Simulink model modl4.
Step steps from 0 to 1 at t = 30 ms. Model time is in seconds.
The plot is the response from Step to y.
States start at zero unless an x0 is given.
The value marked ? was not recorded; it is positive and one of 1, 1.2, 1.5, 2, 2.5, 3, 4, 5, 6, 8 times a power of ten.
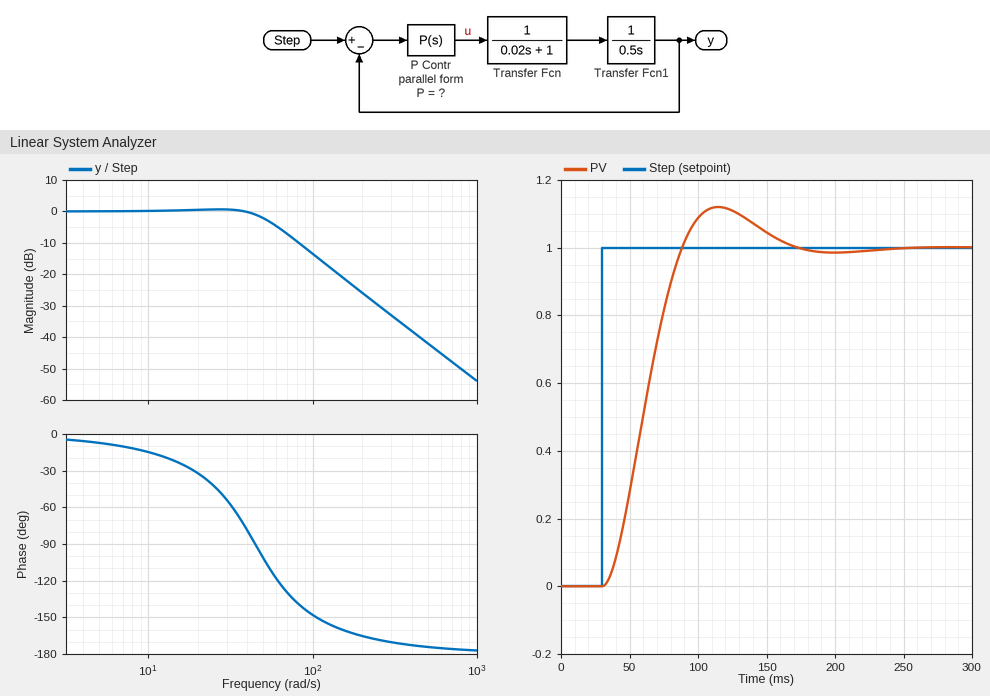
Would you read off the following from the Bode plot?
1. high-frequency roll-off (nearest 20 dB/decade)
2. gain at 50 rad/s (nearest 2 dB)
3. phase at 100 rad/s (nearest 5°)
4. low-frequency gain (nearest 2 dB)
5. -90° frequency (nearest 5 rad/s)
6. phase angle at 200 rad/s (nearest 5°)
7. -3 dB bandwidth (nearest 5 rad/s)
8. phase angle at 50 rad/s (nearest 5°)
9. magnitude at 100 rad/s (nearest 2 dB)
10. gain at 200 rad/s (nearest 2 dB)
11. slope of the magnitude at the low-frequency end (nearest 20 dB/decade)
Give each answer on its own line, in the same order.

-40 dB/decade
-2 dB
-150°
0 dB
45 rad/s
-165°
55 rad/s
-100°
-14 dB
-26 dB
0 dB/decade
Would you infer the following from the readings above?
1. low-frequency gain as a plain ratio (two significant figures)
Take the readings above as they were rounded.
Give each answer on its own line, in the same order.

1.0
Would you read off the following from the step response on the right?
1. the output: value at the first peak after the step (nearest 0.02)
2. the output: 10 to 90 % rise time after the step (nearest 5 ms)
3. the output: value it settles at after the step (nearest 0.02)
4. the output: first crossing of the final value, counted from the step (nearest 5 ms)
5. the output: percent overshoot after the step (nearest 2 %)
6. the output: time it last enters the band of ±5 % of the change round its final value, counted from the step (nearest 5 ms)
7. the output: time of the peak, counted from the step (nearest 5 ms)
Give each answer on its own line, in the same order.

1.12
40 ms
1.00
60 ms
12 %
120 ms
85 ms
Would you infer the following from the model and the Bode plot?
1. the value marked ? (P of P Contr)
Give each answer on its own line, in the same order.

20
